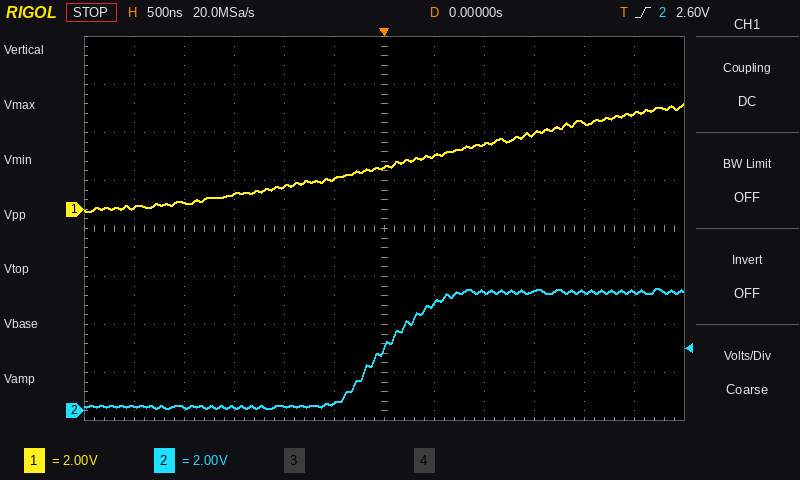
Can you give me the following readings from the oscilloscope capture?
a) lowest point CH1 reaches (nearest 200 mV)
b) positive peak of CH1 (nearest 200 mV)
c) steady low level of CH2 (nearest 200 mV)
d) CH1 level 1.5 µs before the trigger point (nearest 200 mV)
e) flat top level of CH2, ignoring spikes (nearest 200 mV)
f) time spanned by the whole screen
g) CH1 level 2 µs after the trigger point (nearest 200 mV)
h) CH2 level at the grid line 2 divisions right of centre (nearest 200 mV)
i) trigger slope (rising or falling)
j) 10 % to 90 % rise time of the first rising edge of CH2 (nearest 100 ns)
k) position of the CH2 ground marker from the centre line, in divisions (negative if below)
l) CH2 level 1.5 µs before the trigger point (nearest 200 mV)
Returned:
0.0 V
4.4 V
200 mV
600 mV
5.0 V
6 µs
3.6 V
5.0 V
rising
900 ns
-3.8 div
200 mV
